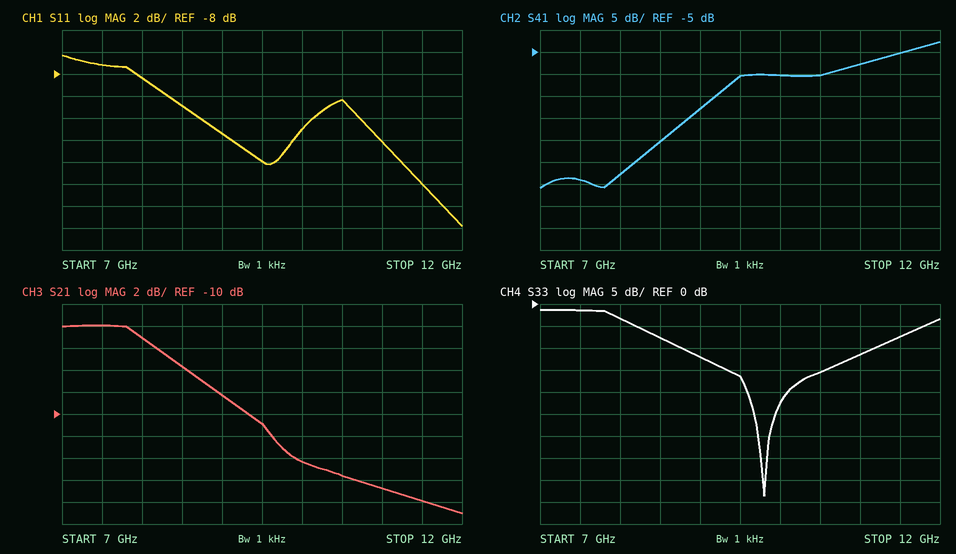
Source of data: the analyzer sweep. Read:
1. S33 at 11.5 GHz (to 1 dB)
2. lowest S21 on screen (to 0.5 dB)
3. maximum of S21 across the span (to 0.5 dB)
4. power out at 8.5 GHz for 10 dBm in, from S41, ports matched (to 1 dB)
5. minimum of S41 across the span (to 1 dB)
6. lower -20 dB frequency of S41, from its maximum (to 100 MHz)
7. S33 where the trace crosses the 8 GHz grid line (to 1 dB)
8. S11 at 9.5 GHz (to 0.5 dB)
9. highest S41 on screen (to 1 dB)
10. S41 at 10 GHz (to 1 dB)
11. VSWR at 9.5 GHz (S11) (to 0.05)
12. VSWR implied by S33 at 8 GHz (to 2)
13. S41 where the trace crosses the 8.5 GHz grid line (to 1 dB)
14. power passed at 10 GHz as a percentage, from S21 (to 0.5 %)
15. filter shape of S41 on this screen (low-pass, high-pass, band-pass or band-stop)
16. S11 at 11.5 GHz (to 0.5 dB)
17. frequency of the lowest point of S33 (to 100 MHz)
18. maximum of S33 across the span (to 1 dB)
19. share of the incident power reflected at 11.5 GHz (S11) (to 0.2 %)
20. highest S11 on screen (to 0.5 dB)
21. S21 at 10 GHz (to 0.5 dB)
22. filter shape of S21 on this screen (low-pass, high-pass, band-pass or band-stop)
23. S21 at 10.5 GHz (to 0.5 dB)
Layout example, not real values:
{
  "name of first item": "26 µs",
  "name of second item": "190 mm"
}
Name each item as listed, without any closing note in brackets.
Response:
{
  "S33 at 11.5 GHz": "-7 dB",
  "lowest S21 on screen": "-19.0 dB",
  "maximum of S21 across the span": "-2.0 dB",
  "power out at 8.5 GHz for 10 dBm in, from S41, ports matched": "-15 dBm",
  "minimum of S41 across the span": "-36 dB",
  "lower -20 dB frequency of S41, from its maximum": "8.7 GHz",
  "S33 where the trace crosses the 8 GHz grid line": "-3 dB",
  "S11 at 9.5 GHz": "-16.0 dB",
  "highest S41 on screen": "-3 dB",
  "S41 at 10 GHz": "-10 dB",
  "VSWR at 9.5 GHz (S11)": "1.40",
  "VSWR implied by S33 at 8 GHz": "6",
  "S41 where the trace crosses the 8.5 GHz grid line": "-25 dB",
  "power passed at 10 GHz as a percentage, from S21": "3.5 %",
  "filter shape of S41 on this screen": "high-pass",
  "S11 at 11.5 GHz": "-18.0 dB",
  "frequency of the lowest point of S33": "9.8 GHz",
  "maximum of S33 across the span": "-1 dB",
  "share of the incident power reflected at 11.5 GHz (S11)": "1.6 %",
  "highest S11 on screen": "-6.5 dB",
  "S21 at 10 GHz": "-14.5 dB",
  "filter shape of S21 on this screen": "low-pass",
  "S21 at 10.5 GHz": "-15.5 dB"
}
